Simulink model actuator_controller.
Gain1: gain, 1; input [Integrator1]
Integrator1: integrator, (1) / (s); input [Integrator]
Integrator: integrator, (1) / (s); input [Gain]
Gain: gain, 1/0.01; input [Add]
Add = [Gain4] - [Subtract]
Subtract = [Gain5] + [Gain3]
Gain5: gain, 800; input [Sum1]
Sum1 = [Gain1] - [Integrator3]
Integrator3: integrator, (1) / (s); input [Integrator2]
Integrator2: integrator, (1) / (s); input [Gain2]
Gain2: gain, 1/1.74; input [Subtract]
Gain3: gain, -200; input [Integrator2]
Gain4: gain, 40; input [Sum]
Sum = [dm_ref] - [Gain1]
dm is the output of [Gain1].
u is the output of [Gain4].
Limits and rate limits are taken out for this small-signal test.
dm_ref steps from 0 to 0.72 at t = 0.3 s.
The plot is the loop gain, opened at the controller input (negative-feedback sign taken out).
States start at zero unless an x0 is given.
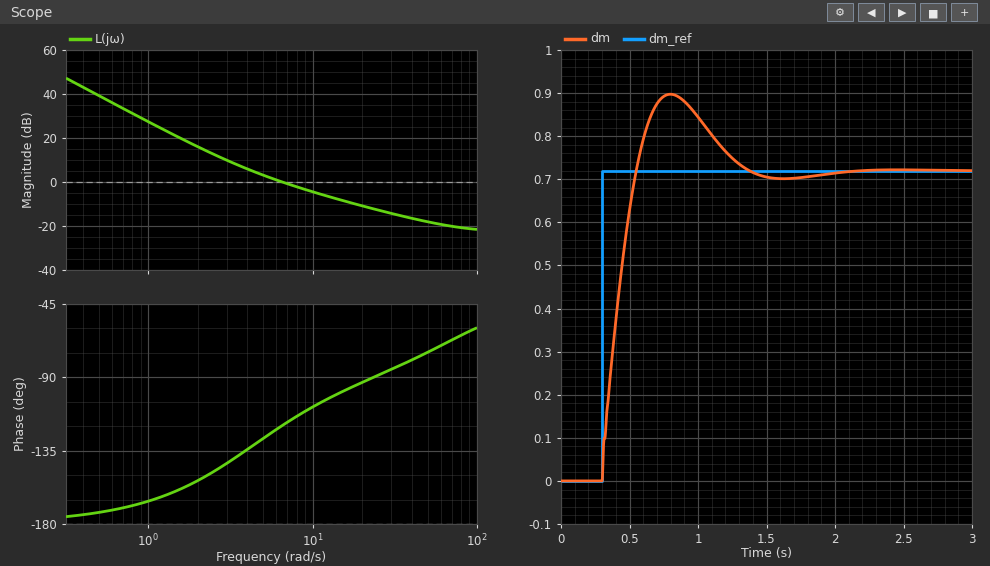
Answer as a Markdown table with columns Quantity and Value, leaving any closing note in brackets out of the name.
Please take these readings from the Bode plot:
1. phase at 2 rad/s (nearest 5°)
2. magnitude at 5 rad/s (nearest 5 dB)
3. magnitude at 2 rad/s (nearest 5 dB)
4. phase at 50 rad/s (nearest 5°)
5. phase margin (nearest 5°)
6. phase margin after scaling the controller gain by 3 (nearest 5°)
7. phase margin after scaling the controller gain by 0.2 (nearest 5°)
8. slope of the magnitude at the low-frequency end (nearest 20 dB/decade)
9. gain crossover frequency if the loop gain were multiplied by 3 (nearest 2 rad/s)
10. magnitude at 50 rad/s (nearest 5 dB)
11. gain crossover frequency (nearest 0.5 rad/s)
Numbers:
| Quantity | Value |
|---|---|
| phase at 2 rad/s | -155° |
| magnitude at 5 rad/s | 5 dB |
| magnitude at 2 rad/s | 15 dB |
| phase at 50 rad/s | -75° |
| phase margin | 60° |
| phase margin after scaling the controller gain by 3 | 85° |
| phase margin after scaling the controller gain by 0.2 | 30° |
| slope of the magnitude at the low-frequency end | -40 dB/decade |
| gain crossover frequency if the loop gain were multiplied by 3 | 18 rad/s |
| magnitude at 50 rad/s | -20 dB |
| gain crossover frequency | 6.5 rad/s |
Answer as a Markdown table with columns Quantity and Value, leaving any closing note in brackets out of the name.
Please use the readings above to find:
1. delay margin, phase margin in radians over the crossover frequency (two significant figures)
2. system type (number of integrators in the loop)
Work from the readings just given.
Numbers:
| Quantity | Value |
|---|---|
| delay margin, phase margin in radians over the crossover frequency | 0.16 s |
| system type | 2 |
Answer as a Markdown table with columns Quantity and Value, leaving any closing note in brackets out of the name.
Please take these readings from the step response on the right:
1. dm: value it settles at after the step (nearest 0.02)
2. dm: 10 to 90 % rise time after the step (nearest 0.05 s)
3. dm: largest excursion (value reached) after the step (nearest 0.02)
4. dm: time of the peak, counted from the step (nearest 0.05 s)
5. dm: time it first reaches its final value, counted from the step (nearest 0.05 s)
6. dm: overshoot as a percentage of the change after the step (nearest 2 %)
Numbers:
| Quantity | Value |
|---|---|
| dm: value it settles at after the step | 0.72 |
| dm: 10 to 90 % rise time after the step | 0.20 s |
| dm: largest excursion (value reached) after the step | 0.90 |
| dm: time of the peak, counted from the step | 0.50 s |
| dm: time it first reaches its final value, counted from the step | 0.25 s |
| dm: overshoot as a percentage of the change after the step | 24 % |
